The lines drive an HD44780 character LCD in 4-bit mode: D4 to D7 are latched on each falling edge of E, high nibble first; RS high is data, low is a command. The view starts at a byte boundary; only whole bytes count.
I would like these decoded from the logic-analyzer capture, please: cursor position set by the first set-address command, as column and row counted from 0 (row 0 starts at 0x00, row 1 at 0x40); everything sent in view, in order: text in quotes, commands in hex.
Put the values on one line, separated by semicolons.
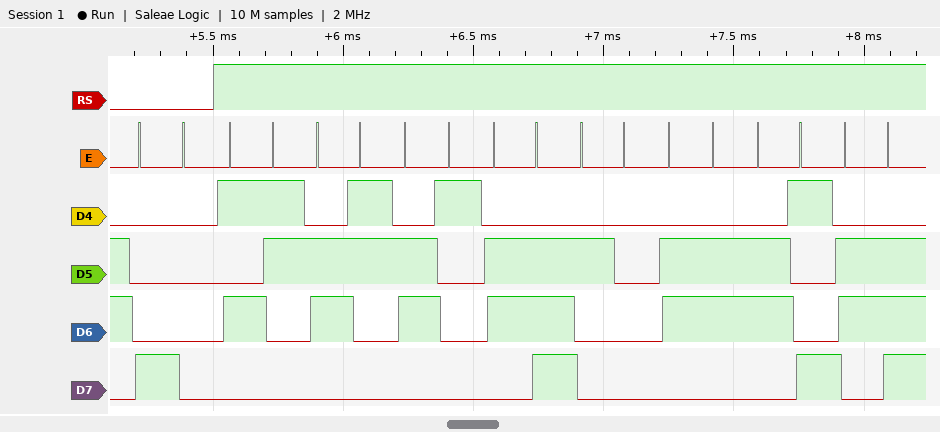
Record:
column 0, row 0; 0x80 "Scan fin"
